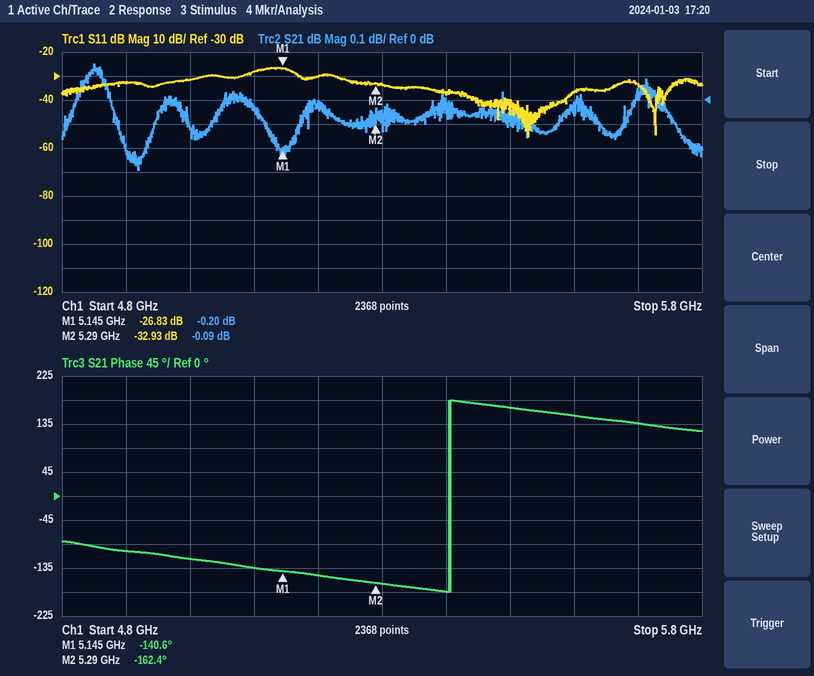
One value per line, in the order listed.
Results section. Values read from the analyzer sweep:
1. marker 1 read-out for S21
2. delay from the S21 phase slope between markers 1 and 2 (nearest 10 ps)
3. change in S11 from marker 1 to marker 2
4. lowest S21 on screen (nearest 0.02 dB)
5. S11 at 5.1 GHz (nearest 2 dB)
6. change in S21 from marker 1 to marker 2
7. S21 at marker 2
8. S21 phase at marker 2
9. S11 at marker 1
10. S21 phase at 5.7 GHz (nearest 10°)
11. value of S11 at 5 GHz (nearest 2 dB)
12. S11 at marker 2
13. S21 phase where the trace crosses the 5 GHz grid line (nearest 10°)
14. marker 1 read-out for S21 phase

-0.20 dB
420 ps
-6.10 dB
-0.30 dB
-28 dB
0.11 dB
-0.09 dB
-162.4°
-26.83 dB
140°
-32 dB
-32.93 dB
-120°
-140.6°
